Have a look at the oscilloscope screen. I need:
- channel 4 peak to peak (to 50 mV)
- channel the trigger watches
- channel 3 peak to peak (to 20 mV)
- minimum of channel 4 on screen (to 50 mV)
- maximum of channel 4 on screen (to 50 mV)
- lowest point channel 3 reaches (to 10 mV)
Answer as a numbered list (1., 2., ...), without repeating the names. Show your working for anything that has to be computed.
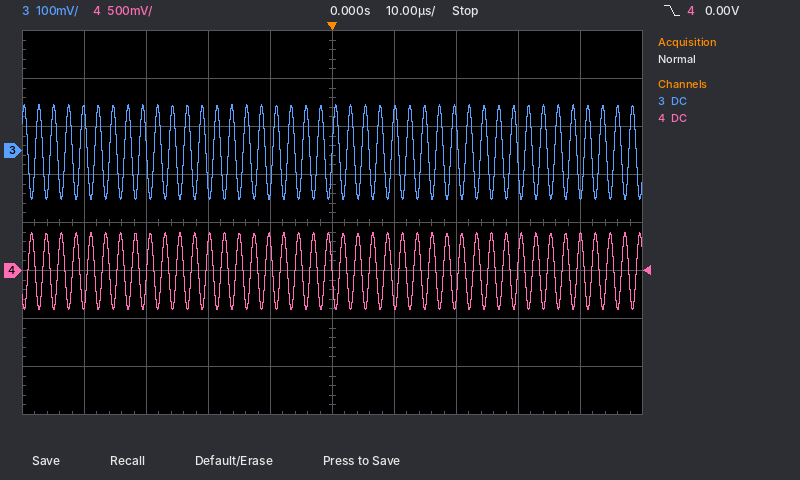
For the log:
1. 400 mV − (-400 mV) = 800 mV
2. channel 4
3. 200 mV
4. -400 mV
5. 400 mV
6. -100 mV
